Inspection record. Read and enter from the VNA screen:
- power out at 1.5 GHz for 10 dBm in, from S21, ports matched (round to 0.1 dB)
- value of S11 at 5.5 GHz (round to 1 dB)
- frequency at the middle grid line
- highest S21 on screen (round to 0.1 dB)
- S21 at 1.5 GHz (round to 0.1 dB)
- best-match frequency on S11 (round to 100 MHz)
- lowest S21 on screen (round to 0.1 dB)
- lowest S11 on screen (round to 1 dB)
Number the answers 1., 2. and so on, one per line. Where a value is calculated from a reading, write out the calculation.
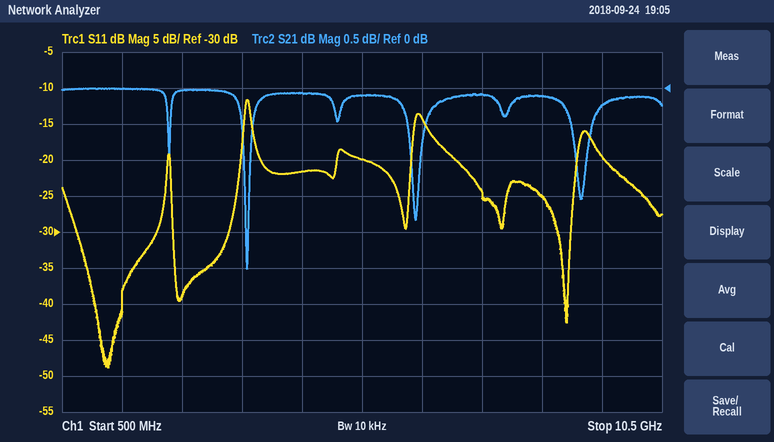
1. 10 dBm + (0.0 dB) = 10.0 dBm
2. -20 dB
3. 5.5 GHz
4. 0.0 dB
5. 0.0 dB
6. 1.3 GHz
7. -2.5 dB
8. -49 dB
